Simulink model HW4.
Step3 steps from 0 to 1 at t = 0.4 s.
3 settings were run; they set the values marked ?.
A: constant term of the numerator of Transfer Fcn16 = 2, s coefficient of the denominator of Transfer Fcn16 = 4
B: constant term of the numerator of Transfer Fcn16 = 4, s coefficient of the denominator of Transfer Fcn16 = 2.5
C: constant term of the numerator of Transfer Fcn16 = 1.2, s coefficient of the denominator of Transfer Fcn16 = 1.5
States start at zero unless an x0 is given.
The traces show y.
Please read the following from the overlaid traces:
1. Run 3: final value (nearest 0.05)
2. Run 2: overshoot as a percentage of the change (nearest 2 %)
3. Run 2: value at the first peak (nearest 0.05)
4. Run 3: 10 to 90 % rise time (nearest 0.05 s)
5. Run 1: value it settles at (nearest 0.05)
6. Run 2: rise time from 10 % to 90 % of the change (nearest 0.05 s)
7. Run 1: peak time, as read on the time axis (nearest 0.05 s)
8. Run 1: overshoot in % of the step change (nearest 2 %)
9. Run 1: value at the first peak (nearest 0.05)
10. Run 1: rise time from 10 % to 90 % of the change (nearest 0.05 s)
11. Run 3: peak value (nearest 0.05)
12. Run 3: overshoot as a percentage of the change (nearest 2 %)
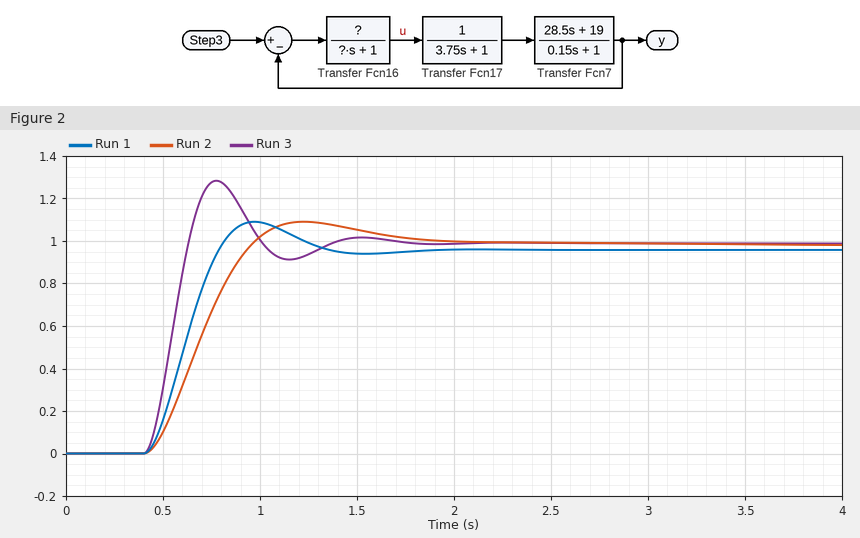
1.00
12 %
1.10
0.15 s
0.95
0.35 s
0.95 s
14 %
1.10
0.25 s
1.30
30 %
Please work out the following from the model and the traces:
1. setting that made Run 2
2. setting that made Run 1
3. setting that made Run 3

A
C
B
